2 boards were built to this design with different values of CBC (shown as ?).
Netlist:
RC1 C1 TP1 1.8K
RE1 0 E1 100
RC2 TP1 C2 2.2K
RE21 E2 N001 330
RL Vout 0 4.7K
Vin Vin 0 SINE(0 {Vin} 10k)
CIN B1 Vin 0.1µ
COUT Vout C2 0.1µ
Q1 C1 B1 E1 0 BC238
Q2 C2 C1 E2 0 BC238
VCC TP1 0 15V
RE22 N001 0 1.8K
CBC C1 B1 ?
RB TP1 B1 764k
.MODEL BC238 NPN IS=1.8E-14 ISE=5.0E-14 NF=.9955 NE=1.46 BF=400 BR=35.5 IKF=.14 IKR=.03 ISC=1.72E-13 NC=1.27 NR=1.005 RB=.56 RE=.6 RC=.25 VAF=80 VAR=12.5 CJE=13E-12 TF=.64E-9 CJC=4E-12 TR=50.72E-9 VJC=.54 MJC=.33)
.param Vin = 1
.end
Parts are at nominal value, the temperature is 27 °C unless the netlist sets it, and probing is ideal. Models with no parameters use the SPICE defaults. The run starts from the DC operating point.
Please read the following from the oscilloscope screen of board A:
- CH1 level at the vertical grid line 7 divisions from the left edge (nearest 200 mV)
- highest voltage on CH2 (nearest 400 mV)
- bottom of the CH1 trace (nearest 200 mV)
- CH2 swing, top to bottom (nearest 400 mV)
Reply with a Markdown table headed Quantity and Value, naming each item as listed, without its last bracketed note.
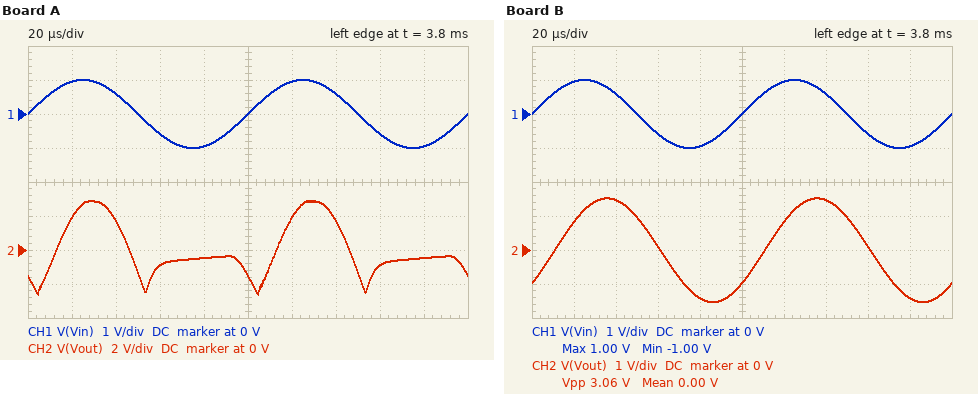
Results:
| Quantity | Value |
|---|---|
| CH1 level at the vertical grid line 7 divisions from the left edge | 600 mV |
| highest voltage on CH2 | 2.8 V |
| bottom of the CH1 trace | -1.0 V |
| CH2 swing, top to bottom | 5.6 V |
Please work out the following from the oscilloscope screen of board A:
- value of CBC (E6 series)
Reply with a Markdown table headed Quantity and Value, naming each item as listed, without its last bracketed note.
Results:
| Quantity | Value |
|---|---|
| value of CBC | 4.7 nF |
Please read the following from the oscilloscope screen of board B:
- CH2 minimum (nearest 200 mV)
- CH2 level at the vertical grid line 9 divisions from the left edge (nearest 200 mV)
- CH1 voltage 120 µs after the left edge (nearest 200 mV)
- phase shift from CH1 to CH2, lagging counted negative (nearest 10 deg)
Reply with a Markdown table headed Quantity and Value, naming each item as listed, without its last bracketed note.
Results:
| Quantity | Value |
|---|---|
| CH2 minimum | -1.6 V |
| CH2 level at the vertical grid line 9 divisions from the left edge | -1.4 V |
| CH1 voltage 120 µs after the left edge | 1.0 V |
| phase shift from CH1 to CH2, lagging counted negative | -40 deg |
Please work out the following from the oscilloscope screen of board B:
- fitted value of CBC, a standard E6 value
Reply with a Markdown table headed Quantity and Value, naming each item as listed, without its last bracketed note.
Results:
| Quantity | Value |
|---|---|
| fitted value of CBC, a standard E6 value | 33 nF |
